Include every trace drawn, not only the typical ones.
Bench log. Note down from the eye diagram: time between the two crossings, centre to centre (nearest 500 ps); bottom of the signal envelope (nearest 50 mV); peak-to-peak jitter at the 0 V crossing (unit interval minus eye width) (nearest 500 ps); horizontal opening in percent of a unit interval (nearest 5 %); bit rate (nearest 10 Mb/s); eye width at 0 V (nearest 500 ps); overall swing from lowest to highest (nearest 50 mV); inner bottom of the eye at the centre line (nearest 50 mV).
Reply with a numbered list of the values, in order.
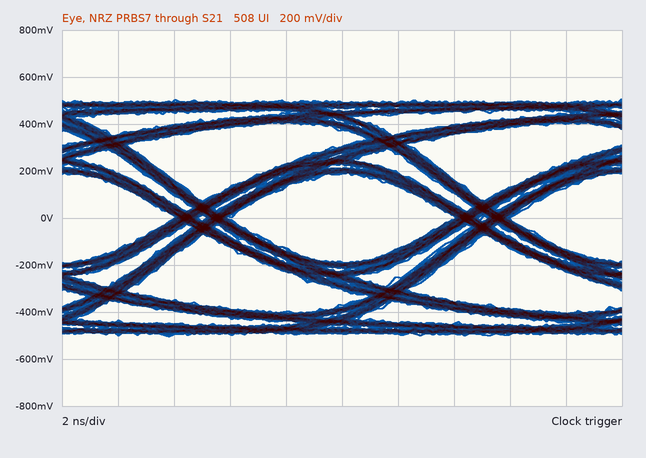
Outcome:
1. 10.0 ns
2. -500 mV
3. 2.0 ns
4. 80 %
5. 100 Mb/s
6. 8.0 ns
7. 1.00 V
8. -200 mV
